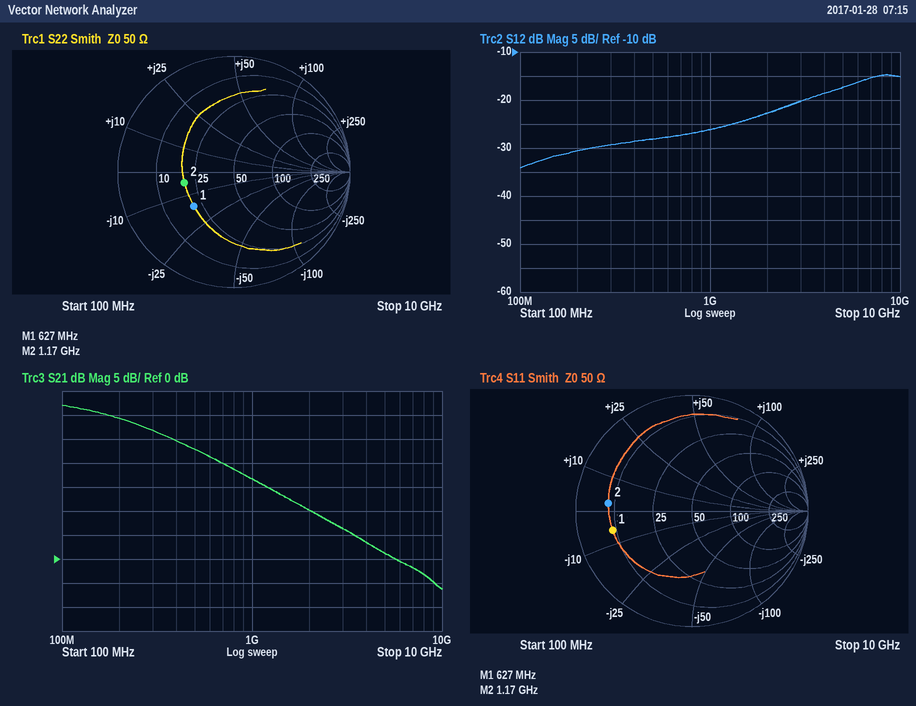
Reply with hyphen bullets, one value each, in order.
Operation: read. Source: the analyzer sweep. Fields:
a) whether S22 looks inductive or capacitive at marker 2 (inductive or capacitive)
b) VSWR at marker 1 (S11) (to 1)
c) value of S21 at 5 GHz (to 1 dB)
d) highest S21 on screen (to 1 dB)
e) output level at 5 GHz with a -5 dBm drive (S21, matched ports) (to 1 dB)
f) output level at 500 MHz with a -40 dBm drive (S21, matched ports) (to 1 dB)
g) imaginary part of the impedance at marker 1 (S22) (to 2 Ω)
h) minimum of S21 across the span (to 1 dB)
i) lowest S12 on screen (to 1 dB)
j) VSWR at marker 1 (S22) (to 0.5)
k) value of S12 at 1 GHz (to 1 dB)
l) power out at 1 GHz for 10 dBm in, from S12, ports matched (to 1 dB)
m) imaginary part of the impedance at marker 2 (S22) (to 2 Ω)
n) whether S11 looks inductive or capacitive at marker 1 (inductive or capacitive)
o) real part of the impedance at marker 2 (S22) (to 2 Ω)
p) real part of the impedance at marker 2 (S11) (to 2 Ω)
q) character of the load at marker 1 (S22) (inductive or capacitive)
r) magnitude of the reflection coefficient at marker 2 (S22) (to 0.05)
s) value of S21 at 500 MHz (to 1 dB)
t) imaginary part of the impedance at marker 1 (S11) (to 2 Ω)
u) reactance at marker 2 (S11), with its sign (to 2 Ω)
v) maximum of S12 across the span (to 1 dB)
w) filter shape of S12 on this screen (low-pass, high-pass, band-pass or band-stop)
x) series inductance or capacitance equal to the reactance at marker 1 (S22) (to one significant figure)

- capacitive
- 6
- 1 dB
- 32 dB
- -4 dBm
- -17 dBm
- -16 Ω
- -6 dB
- -34 dB
- 2.5
- -26 dB
- -16 dBm
- -4 Ω
- capacitive
- 20 Ω
- 8 Ω
- capacitive
- 0.45
- 23 dB
- -6 Ω
- +2 Ω
- -15 dB
- high-pass
- 20 pF
